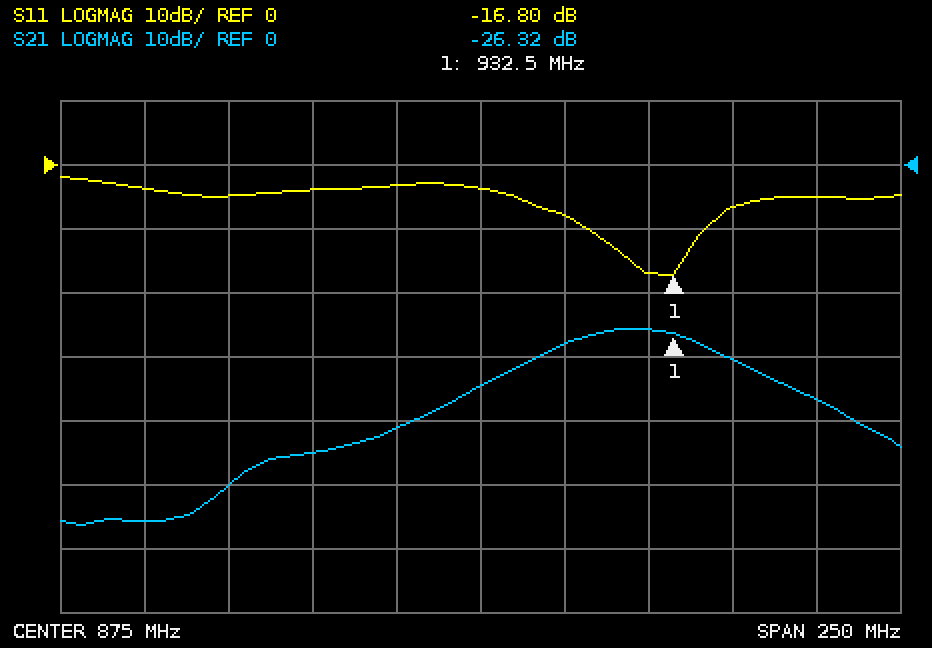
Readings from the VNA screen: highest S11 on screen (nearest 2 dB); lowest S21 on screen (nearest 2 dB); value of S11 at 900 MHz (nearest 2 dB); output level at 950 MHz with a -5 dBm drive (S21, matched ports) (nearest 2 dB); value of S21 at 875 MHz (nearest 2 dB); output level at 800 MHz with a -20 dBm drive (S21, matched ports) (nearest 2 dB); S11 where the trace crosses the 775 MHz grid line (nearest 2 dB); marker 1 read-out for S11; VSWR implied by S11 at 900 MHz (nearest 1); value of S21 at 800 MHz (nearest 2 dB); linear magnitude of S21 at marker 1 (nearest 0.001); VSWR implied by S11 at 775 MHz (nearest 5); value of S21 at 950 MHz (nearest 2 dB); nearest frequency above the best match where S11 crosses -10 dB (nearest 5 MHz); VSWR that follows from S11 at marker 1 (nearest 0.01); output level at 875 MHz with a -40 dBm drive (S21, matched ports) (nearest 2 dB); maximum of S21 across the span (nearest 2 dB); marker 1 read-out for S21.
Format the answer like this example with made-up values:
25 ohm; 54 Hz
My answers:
-2 dB; -56 dB; -8 dB; -36 dBm; -34 dB; -70 dBm; -4 dB; -16.80 dB; 2; -50 dB; 0.048; 5; -30 dB; 940 MHz; 1.34; -74 dBm; -26 dB; -26.32 dB
